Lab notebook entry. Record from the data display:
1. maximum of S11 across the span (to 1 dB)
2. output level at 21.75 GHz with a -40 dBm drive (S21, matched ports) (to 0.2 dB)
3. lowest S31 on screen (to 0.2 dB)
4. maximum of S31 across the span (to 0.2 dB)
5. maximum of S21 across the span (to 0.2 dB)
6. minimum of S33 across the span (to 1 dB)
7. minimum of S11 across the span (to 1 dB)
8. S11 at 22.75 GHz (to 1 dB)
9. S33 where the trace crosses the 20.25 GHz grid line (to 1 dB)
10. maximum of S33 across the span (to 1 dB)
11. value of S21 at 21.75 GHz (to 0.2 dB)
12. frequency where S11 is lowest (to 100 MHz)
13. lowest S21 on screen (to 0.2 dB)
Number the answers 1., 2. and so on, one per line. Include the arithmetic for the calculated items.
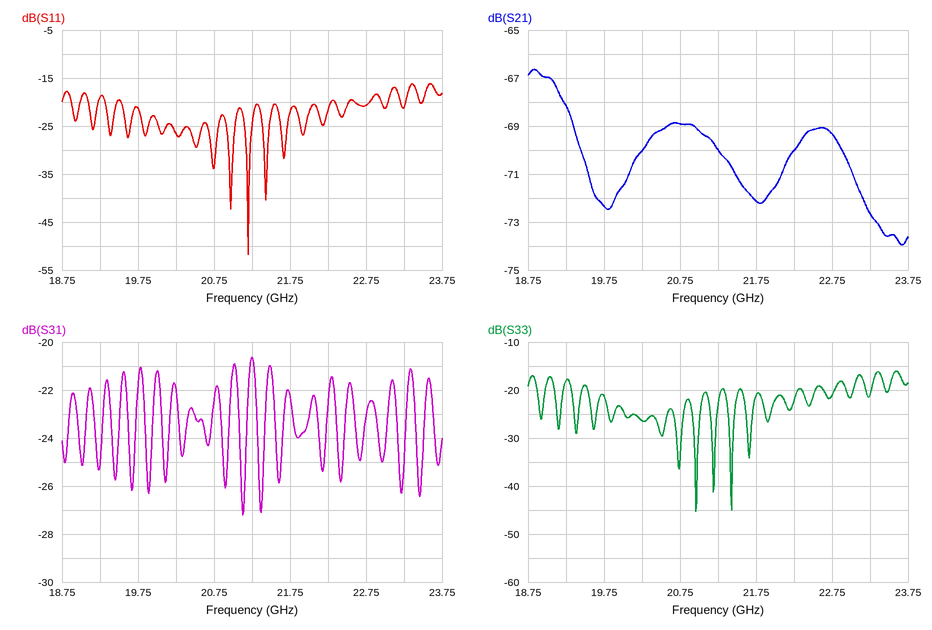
1. -16 dB
2. -40 dBm + (-72.2 dB) = -112.2 dBm
3. -27.2 dB
4. -20.6 dB
5. -66.6 dB
6. -45 dB
7. -52 dB
8. -21 dB
9. -26 dB
10. -16 dB
11. -72.2 dB
12. 21.2 GHz
13. -74.0 dB
